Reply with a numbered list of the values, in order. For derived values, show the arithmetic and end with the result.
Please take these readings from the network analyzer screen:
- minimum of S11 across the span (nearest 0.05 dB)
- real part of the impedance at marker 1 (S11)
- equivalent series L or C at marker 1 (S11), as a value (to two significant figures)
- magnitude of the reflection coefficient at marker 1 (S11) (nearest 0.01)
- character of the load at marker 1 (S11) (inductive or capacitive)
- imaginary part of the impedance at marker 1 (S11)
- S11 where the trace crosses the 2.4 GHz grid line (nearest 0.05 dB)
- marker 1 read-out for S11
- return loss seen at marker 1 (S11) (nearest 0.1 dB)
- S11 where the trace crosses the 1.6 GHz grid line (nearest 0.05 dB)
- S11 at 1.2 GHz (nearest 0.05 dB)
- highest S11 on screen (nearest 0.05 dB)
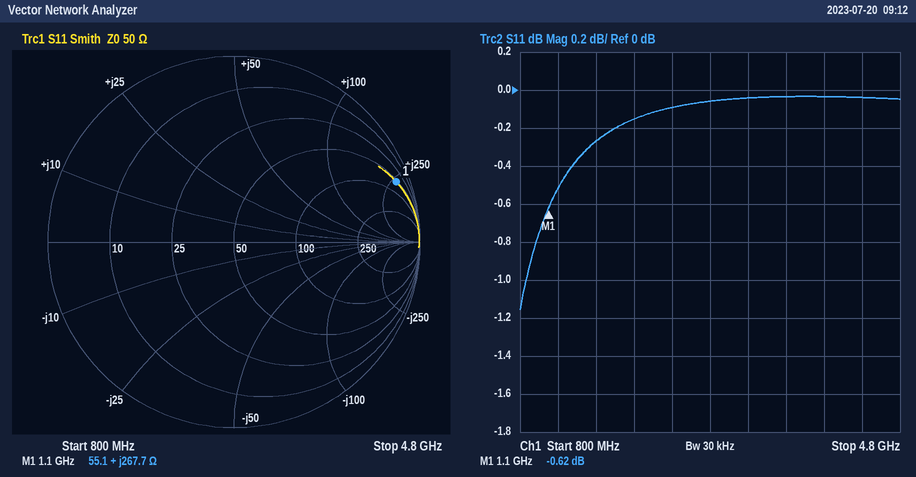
1. -1.15 dB
2. 55.1 Ω
3. L = 267.7 Ω/(2π × 1.1 GHz) ≈ 39 nH
4. 10^(-0.62/20) ≈ 0.93
5. inductive
6. +267.7 Ω
7. -0.10 dB
8. -0.62 dB
9. 0.6 dB
10. -0.25 dB
11. -0.50 dB
12. -0.05 dB
